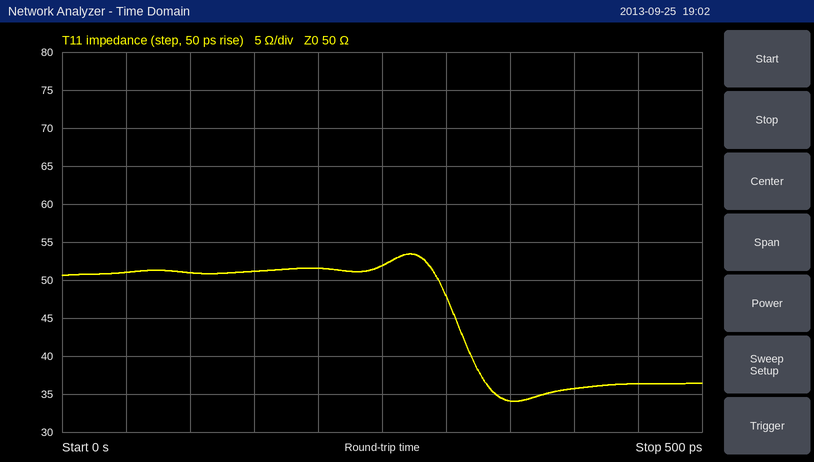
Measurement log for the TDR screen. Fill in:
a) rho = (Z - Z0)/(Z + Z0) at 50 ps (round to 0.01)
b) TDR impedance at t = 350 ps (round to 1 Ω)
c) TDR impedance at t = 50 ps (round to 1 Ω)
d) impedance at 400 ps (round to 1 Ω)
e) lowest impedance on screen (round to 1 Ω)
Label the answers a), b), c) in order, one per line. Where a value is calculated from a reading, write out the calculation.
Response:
a) (51 − 50)/(51 + 50) ≈ +0.01
b) 34 Ω
c) 51 Ω
d) 36 Ω
e) 34 Ω
